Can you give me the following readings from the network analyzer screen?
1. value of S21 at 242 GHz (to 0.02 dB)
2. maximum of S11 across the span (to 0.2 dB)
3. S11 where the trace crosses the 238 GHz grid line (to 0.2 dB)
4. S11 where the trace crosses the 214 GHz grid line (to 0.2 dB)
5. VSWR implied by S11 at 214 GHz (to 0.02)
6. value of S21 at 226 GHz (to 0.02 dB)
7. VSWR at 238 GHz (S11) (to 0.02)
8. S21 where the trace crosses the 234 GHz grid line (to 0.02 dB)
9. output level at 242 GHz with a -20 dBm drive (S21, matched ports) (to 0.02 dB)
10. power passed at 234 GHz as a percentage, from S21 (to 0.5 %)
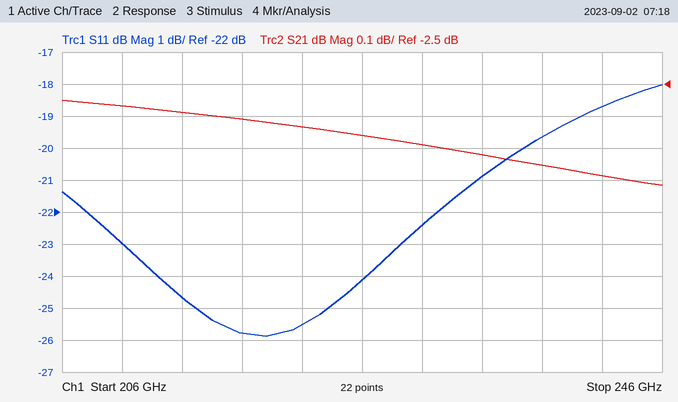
-2.78 dB
-18.0 dB
-19.6 dB
-24.6 dB
1.12
-2.66 dB
1.24
-2.72 dB
-22.78 dBm
53.5 %
